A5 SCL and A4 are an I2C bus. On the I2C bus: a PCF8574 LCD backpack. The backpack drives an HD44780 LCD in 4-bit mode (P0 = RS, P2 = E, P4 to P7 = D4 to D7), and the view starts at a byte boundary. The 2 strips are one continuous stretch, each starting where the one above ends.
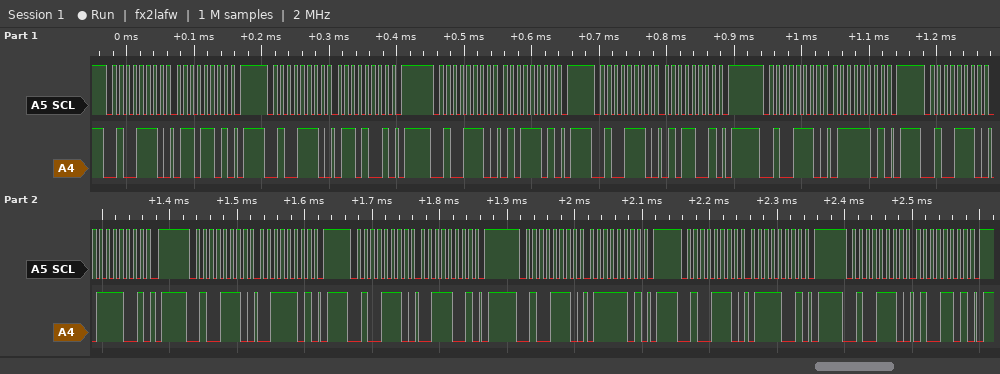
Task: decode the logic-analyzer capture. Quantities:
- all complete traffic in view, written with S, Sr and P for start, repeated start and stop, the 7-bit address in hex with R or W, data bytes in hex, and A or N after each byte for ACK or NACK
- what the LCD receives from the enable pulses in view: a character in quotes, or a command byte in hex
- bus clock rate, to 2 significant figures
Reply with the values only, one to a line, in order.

S 27W A 6D A P S 27W A 69 A P S 27W A 5D A P S 27W A 59 A P S 27W A 7D A P S 27W A 79 A P S 27W A 3D A P S 27W A 39 A P S 27W A 7D A P S 27W A 79 A P S 27W A 4D A P
'e' 's'
100 kHz
